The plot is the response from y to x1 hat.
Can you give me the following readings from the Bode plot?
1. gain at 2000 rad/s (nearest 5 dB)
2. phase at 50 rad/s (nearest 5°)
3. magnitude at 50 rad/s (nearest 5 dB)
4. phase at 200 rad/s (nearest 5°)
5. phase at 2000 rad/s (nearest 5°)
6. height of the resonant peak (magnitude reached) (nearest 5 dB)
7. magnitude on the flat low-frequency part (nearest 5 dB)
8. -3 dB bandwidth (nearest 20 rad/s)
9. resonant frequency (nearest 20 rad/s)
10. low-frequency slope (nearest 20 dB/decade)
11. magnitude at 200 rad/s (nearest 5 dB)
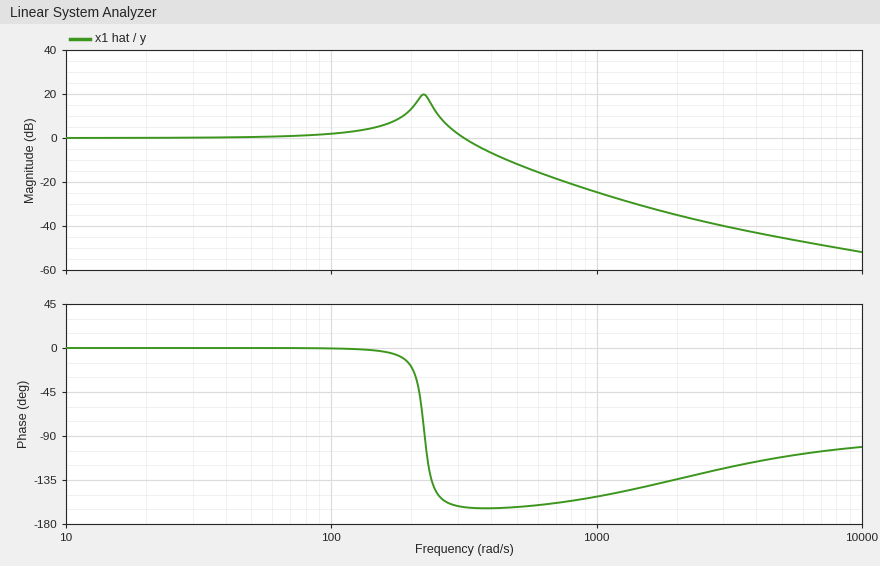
-35 dB
0°
0 dB
-20°
-135°
20 dB
0 dB
340 rad/s
220 rad/s
0 dB/decade
15 dB
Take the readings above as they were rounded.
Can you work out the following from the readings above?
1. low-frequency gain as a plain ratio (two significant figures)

1.0
